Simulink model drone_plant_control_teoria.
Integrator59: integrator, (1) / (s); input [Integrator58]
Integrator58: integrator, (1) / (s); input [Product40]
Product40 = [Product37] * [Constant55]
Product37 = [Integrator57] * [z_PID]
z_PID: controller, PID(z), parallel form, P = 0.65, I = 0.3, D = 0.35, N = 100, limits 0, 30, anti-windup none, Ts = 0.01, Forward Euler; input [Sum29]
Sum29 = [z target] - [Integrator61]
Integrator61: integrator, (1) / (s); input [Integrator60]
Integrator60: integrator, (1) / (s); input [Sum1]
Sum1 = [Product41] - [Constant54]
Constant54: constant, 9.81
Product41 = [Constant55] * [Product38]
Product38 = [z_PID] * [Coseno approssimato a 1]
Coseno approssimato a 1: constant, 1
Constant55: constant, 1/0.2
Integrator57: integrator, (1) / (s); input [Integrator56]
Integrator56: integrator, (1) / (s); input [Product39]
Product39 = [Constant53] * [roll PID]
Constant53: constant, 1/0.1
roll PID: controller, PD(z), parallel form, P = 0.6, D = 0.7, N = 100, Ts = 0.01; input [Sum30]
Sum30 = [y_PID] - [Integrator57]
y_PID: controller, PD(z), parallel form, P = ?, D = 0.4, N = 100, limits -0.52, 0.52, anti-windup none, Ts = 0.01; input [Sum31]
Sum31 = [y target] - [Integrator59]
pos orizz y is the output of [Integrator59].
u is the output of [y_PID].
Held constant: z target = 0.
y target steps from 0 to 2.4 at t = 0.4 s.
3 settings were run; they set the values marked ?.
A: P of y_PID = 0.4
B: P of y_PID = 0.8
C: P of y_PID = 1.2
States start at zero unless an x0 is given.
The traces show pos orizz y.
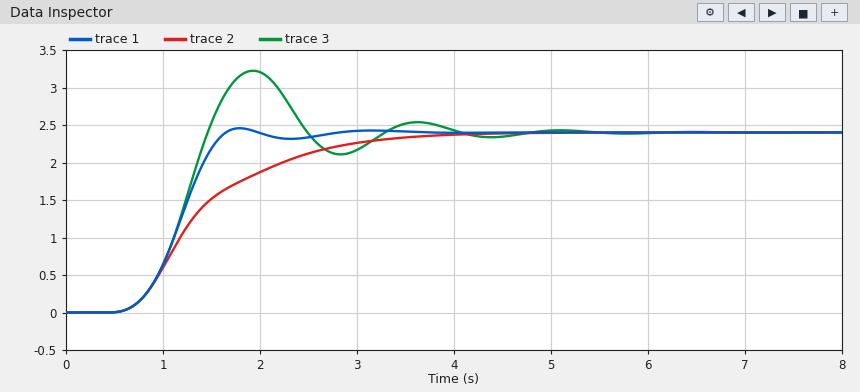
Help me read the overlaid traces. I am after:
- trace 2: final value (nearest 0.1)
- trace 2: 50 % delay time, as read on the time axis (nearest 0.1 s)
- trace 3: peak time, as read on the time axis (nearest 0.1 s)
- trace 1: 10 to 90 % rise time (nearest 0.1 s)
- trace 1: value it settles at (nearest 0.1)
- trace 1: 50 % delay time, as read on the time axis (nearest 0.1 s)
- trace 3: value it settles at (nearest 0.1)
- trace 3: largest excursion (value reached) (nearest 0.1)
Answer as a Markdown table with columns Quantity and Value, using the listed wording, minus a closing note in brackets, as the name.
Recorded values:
| Quantity | Value |
|---|---|
| trace 2: final value | 2.4 |
| trace 2: 50 % delay time, as read on the time axis | 1.3 s |
| trace 3: peak time, as read on the time axis | 1.9 s |
| trace 1: 10 to 90 % rise time | 0.7 s |
| trace 1: value it settles at | 2.4 |
| trace 1: 50 % delay time, as read on the time axis | 1.2 s |
| trace 3: value it settles at | 2.4 |
| trace 3: largest excursion (value reached) | 3.2 |
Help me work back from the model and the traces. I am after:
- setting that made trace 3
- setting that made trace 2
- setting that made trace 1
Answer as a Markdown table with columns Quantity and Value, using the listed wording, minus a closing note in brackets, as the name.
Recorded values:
| Quantity | Value |
|---|---|
| setting that made trace 3 | C |
| setting that made trace 2 | A |
| setting that made trace 1 | B |
